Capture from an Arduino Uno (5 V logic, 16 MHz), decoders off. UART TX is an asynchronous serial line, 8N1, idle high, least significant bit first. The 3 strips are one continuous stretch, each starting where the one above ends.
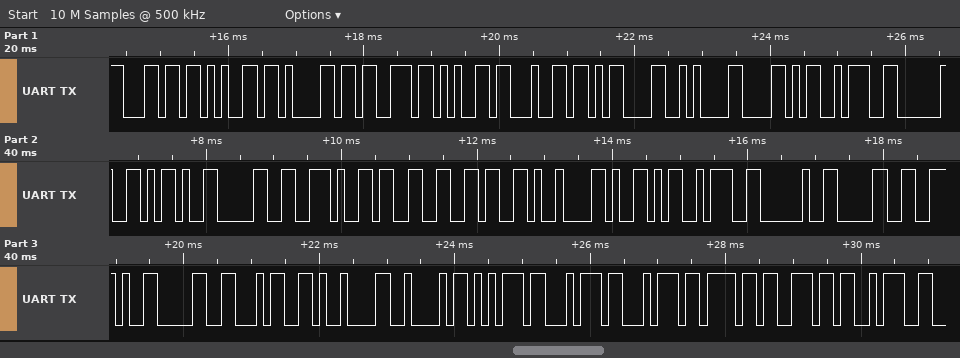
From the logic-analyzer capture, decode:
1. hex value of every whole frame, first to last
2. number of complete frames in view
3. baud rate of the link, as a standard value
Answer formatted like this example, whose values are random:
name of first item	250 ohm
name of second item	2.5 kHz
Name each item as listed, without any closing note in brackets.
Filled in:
hex value of every whole frame, first to last	6C 65 61 73 65 64 0D 0A 58 3A 20 2D 30 2E 33 36 09 59 3A 20 30 2E 30 34 09 42 75 74 74 6F 6E 3A
number of complete frames in view	32
baud rate of the link, as a standard value	9600 baud
